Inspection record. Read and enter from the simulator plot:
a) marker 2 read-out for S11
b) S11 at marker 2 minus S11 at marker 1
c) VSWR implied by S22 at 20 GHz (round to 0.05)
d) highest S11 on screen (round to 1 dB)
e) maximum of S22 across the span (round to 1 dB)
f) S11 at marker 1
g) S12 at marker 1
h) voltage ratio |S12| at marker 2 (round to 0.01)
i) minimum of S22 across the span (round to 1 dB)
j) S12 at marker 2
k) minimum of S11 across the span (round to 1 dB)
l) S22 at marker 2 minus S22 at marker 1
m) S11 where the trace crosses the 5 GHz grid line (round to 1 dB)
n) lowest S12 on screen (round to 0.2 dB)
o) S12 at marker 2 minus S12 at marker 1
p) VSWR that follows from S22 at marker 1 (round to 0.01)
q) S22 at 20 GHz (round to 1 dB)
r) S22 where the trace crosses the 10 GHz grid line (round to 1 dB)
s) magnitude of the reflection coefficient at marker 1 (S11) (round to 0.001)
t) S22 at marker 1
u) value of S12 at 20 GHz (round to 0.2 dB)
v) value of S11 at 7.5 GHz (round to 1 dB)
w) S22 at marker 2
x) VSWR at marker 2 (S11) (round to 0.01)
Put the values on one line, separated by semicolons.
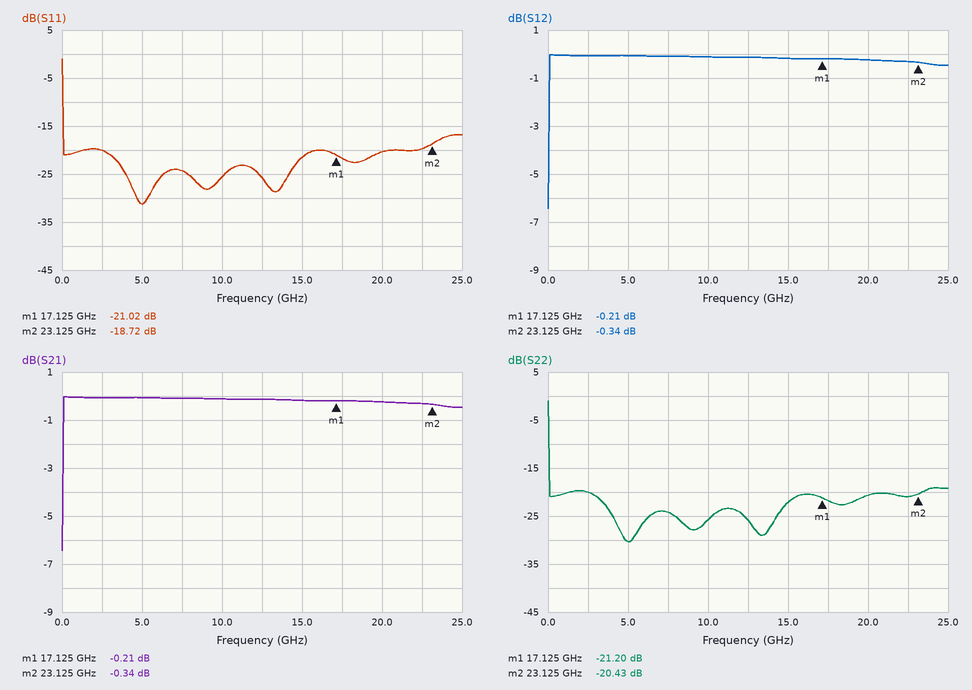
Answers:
-18.72 dB; 2.30 dB; 1.20; -1 dB; -1 dB; -21.02 dB; -0.21 dB; 0.96; -30 dB; -0.34 dB; -31 dB; 0.77 dB; -31 dB; -6.4 dB; -0.13 dB; 1.19; -21 dB; -26 dB; 0.089; -21.20 dB; -0.2 dB; -24 dB; -20.43 dB; 1.26
